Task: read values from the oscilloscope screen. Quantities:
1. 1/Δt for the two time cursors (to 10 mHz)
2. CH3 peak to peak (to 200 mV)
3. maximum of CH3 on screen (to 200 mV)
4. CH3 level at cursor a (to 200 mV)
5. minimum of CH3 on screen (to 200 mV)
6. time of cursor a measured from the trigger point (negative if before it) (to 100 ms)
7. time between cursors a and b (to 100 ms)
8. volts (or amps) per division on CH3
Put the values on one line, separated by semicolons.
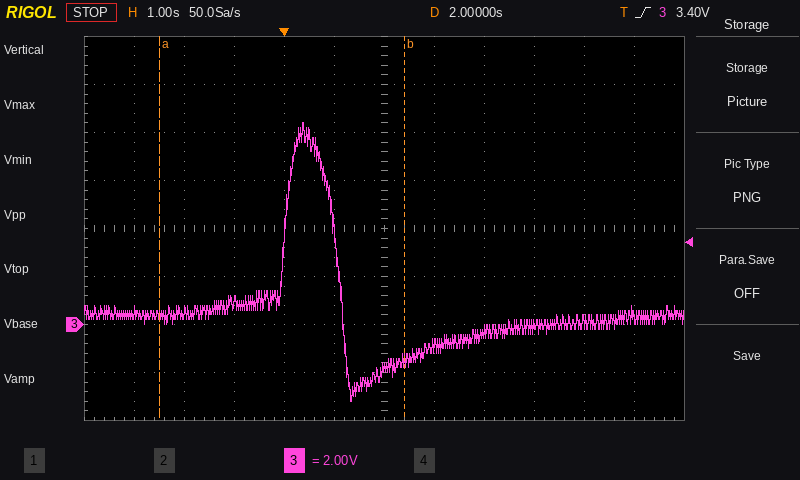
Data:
200 mHz; 11.6 V; 8.4 V; 400 mV; -3.2 V; -2.5 s; 4.9 s; 2 V
